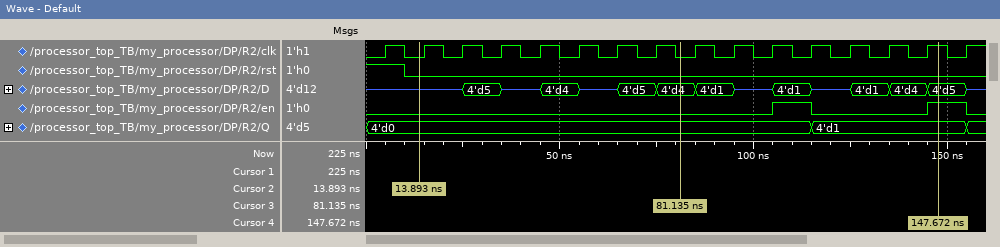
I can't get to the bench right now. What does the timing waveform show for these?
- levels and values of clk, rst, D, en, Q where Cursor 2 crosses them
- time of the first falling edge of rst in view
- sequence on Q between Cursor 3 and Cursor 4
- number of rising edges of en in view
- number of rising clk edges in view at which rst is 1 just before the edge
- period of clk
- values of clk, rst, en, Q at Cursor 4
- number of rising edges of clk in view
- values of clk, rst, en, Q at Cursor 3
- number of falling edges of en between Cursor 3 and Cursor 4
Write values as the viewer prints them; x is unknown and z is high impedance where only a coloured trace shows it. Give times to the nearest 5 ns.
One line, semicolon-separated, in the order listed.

clk=0, rst=0, D=z, en=0, Q=4'd0; 10 ns; 4'd0, 4'd1; 2; 1; 10 ns; clk=1, rst=0, en=1, Q=4'd1; 16; clk=0, rst=0, en=0, Q=4'd0; 1
